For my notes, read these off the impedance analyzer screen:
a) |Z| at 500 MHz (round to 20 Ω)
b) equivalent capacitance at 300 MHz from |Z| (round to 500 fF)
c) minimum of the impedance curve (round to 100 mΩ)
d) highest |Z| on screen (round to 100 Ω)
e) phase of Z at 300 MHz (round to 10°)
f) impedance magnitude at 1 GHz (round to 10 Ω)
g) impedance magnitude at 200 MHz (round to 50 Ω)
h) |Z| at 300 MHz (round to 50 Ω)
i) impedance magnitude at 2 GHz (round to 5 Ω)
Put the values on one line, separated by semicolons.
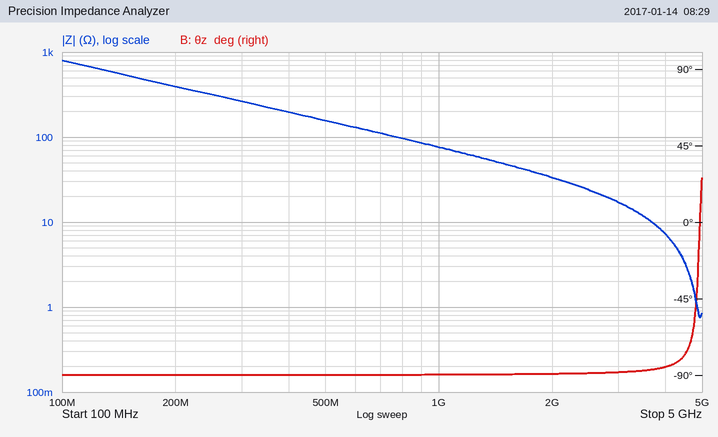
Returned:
160 Ω; 2.0 pF; 800 mΩ; 800 Ω; -90°; 80 Ω; 400 Ω; 250 Ω; 35 Ω
